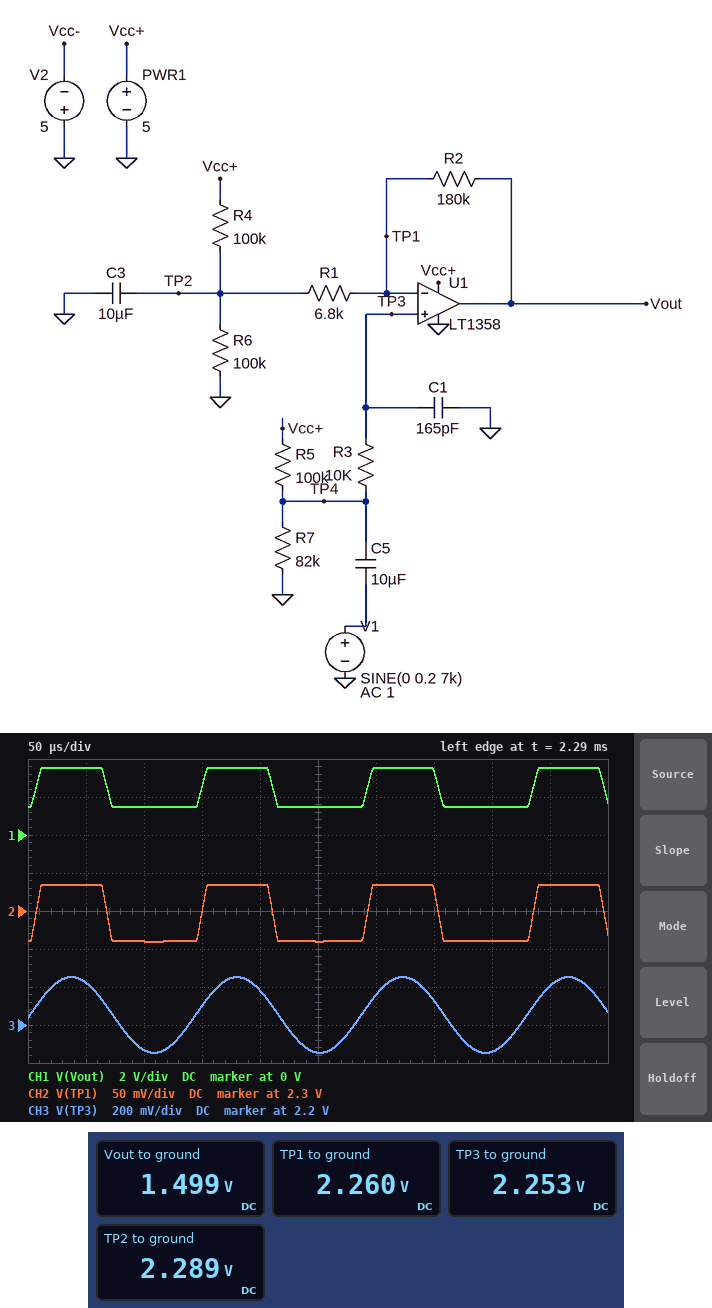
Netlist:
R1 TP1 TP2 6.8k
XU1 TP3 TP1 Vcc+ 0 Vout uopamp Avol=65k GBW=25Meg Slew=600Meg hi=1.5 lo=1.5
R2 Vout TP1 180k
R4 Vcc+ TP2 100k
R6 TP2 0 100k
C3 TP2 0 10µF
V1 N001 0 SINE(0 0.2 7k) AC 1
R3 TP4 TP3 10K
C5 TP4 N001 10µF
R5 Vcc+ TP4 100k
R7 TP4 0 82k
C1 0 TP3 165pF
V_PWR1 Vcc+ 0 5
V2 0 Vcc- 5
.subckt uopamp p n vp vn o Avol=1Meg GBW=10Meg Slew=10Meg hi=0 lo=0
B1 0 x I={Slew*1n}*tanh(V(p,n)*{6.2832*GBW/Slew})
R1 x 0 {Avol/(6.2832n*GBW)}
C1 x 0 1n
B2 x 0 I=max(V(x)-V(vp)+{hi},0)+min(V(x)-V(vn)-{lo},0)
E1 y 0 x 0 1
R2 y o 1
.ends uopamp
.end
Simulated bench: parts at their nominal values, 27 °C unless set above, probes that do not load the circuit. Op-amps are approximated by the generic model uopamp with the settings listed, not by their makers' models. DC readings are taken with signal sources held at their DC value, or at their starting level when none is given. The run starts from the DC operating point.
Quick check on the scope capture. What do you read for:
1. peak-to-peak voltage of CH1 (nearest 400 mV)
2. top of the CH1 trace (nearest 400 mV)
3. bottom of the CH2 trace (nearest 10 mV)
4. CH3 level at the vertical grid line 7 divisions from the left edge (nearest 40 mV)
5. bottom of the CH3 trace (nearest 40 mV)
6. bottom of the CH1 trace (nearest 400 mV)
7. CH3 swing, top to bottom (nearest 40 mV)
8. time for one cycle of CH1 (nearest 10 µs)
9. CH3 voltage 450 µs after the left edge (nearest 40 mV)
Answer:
2.0 V
3.6 V
2.26 V
2.32 V
2.04 V
1.6 V
400 mV
140 µs
2.40 V
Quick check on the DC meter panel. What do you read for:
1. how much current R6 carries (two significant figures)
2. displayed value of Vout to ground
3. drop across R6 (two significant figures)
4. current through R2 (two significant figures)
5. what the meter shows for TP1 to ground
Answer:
23 µA
1.499 V
2.3 V
4.2 µA
2.260 V
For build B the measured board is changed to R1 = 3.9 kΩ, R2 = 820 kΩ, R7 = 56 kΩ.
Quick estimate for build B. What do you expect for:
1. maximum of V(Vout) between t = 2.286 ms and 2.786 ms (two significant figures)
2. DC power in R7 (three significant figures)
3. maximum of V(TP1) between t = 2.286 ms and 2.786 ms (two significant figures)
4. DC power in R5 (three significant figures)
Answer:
1.4 V
57.5 µW
2.4 V
103 µW
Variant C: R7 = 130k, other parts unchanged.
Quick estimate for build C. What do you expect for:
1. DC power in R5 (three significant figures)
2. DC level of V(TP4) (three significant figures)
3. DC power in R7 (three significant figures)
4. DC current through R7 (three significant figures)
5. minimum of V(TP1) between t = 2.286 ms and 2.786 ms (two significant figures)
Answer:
47.3 µW
2.83 V
61.4 µW
21.7 µA
2.7 V
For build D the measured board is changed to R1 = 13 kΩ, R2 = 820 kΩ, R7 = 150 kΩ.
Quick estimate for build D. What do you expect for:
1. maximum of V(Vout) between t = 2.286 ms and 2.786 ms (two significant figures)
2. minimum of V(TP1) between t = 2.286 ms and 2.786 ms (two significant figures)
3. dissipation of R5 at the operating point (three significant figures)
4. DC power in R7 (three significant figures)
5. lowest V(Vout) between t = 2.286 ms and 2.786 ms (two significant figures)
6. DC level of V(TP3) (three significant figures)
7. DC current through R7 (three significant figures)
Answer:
3.6 V
2.6 V
40.0 µW
60.0 µW
3.5 V
3.00 V
20.0 µA
